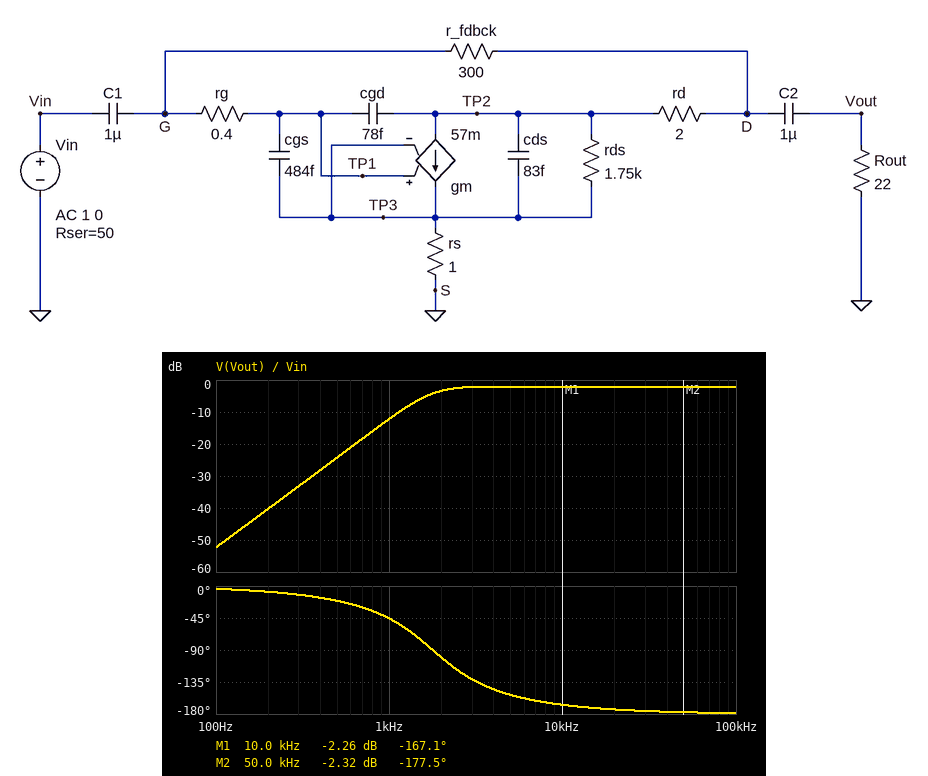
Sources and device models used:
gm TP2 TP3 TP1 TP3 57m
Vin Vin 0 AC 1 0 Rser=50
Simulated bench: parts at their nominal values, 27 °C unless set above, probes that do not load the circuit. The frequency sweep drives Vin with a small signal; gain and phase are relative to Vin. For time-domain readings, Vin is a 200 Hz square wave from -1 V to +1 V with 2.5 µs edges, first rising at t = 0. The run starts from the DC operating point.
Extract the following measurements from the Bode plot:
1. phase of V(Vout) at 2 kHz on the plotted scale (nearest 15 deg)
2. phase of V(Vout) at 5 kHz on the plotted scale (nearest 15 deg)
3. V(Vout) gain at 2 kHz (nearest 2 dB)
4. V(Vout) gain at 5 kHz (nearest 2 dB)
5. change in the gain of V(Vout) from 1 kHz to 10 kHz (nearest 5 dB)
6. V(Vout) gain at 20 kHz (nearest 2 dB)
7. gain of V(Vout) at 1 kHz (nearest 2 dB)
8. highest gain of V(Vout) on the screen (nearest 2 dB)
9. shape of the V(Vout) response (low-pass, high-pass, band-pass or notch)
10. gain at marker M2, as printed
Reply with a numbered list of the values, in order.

1. -105 deg
2. -150 deg
3. -4 dB
4. -2 dB
5. 10 dB
6. -2 dB
7. -12 dB
8. -2 dB
9. high-pass
10. -2.32 dB
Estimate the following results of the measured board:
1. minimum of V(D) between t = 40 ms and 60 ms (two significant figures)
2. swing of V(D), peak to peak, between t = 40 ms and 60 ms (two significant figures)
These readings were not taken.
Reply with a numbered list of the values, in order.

1. -3.2 V
2. 6.3 V
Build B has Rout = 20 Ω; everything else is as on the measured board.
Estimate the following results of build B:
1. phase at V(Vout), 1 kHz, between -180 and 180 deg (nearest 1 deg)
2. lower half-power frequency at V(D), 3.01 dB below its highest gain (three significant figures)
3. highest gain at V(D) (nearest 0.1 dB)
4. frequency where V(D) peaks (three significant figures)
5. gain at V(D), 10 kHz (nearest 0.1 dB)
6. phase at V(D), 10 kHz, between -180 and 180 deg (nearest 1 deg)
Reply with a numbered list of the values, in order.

1. -45 deg
2. 1.02 kHz
3. 8.3 dB
4. 1.83 kHz
5. -0.8 dB
6. 154 deg
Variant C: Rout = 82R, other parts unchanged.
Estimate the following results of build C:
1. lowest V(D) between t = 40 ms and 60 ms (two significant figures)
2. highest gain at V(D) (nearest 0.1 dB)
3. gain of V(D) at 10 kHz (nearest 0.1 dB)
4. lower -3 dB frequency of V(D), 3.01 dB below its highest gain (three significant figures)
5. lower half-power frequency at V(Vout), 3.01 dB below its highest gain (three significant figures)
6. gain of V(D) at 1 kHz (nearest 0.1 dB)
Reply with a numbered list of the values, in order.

1. -3.7 V
2. 6.6 dB
3. 5.5 dB
4. 896 Hz
5. 1.59 kHz
6. 4.3 dB
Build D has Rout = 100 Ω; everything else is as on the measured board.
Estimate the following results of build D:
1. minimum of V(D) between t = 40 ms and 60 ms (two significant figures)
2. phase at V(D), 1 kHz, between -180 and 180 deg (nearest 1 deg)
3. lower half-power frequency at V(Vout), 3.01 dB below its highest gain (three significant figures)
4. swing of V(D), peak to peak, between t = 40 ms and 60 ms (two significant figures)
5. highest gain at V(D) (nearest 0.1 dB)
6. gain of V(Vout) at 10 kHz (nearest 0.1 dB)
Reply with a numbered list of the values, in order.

1. -4.1 V
2. -127 deg
3. 1.60 kHz
4. 8.2 V
5. 6.6 dB
6. 6.2 dB
